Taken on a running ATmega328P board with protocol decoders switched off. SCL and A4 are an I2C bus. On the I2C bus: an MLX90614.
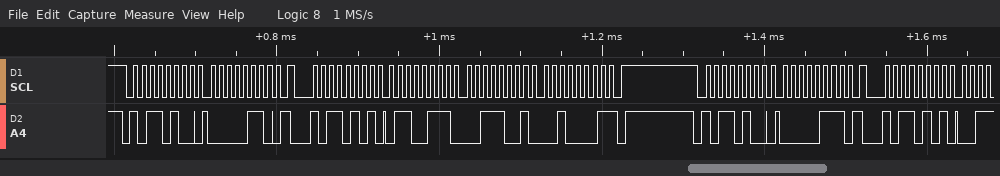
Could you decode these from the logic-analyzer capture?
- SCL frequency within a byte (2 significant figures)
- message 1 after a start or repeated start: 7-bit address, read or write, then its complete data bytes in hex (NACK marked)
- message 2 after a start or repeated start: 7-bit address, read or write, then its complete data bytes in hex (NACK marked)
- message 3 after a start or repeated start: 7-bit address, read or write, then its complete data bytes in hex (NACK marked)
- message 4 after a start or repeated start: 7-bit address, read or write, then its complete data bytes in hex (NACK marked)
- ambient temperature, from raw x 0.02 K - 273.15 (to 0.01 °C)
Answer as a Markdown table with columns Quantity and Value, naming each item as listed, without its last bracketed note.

| Quantity | Value |
|---|---|
| SCL frequency within a byte | 100 kHz |
| message 1 after a start or repeated start: 7-bit address, read or write, then its complete data bytes in hex | 0x5A write: 06 |
| message 2 after a start or repeated start: 7-bit address, read or write, then its complete data bytes in hex | 0x5A read: 67 39 21 NACK |
| message 3 after a start or repeated start: 7-bit address, read or write, then its complete data bytes in hex | 0x5A write: 07 |
| message 4 after a start or repeated start: 7-bit address, read or write, then its complete data bytes in hex | 0x5A read |
| ambient temperature, from raw x 0.02 K - 273.15 | 20.75 °C |
